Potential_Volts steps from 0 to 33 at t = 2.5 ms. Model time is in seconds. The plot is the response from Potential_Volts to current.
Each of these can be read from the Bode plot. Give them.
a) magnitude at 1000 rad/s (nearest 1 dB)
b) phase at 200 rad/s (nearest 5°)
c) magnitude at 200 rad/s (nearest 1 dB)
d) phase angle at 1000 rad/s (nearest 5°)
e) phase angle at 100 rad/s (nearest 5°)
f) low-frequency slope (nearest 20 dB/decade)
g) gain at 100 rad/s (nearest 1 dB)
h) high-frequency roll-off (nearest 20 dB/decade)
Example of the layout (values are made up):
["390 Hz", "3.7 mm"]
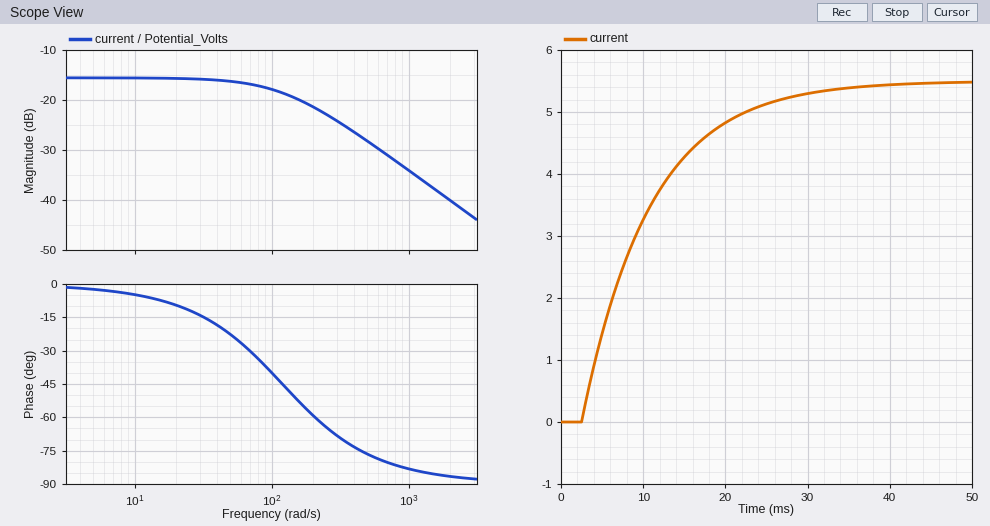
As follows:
["-34 dB", "-60°", "-21 dB", "-85°", "-40°", "0 dB/decade", "-18 dB", "-20 dB/decade"]
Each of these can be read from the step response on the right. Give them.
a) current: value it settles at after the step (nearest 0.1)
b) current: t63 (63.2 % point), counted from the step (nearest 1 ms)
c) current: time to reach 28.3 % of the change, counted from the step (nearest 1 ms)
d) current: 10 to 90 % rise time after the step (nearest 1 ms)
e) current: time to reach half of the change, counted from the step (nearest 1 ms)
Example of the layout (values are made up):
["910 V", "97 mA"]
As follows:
["5.5", "8 ms", "3 ms", "18 ms", "6 ms"]
